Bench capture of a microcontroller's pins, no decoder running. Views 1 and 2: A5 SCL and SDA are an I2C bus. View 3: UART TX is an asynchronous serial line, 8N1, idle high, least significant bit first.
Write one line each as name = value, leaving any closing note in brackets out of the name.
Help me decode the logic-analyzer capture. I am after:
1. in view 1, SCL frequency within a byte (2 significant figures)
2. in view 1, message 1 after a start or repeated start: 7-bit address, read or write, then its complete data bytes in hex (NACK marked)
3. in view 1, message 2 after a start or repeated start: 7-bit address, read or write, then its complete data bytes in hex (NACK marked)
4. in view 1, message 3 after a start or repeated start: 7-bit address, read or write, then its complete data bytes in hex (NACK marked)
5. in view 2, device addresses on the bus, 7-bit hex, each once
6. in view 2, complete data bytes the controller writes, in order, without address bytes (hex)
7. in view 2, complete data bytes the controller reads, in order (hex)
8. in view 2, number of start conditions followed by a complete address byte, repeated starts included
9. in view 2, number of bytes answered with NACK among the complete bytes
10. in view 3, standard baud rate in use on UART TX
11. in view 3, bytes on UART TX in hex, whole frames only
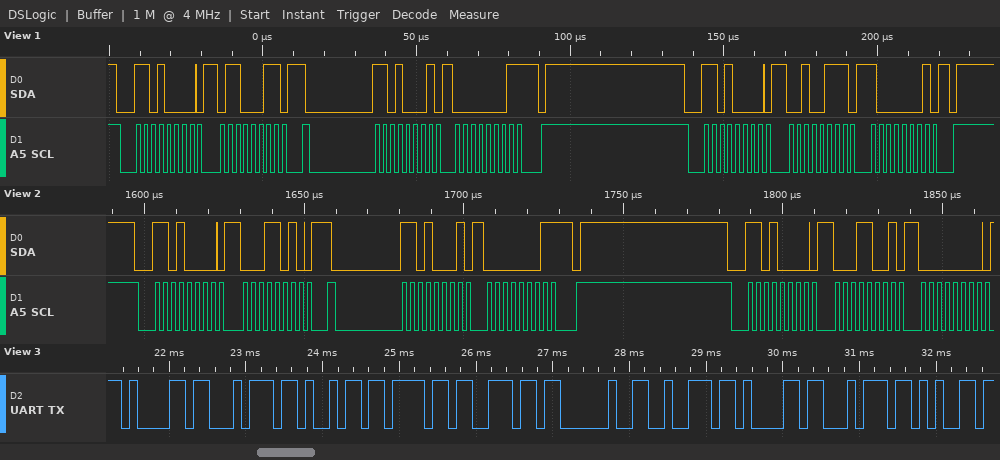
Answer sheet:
in view 1, SCL frequency within a byte = 400 kHz
in view 1, message 1 after a start or repeated start: 7-bit address, read or write, then its complete data bytes in hex = 0x68 write: 63
in view 1, message 2 after a start or repeated start: 7-bit address, read or write, then its complete data bytes in hex = 0x68 read: 01 NACK
in view 1, message 3 after a start or repeated start: 7-bit address, read or write, then its complete data bytes in hex = 0x68 write: 27 81
in view 2, device addresses on the bus, 7-bit hex, each once = 0x68
in view 2, complete data bytes the controller writes, in order, without address bytes = 1A 19 00
in view 2, complete data bytes the controller reads, in order = 01
in view 2, number of start conditions followed by a complete address byte, repeated starts included = 3
in view 2, number of bytes answered with NACK among the complete bytes = 1
in view 3, standard baud rate in use on UART TX = 9600 baud
in view 3, bytes on UART TX in hex, whole frames only = 61 74 69 6F 6E 20 72 61 74 65
